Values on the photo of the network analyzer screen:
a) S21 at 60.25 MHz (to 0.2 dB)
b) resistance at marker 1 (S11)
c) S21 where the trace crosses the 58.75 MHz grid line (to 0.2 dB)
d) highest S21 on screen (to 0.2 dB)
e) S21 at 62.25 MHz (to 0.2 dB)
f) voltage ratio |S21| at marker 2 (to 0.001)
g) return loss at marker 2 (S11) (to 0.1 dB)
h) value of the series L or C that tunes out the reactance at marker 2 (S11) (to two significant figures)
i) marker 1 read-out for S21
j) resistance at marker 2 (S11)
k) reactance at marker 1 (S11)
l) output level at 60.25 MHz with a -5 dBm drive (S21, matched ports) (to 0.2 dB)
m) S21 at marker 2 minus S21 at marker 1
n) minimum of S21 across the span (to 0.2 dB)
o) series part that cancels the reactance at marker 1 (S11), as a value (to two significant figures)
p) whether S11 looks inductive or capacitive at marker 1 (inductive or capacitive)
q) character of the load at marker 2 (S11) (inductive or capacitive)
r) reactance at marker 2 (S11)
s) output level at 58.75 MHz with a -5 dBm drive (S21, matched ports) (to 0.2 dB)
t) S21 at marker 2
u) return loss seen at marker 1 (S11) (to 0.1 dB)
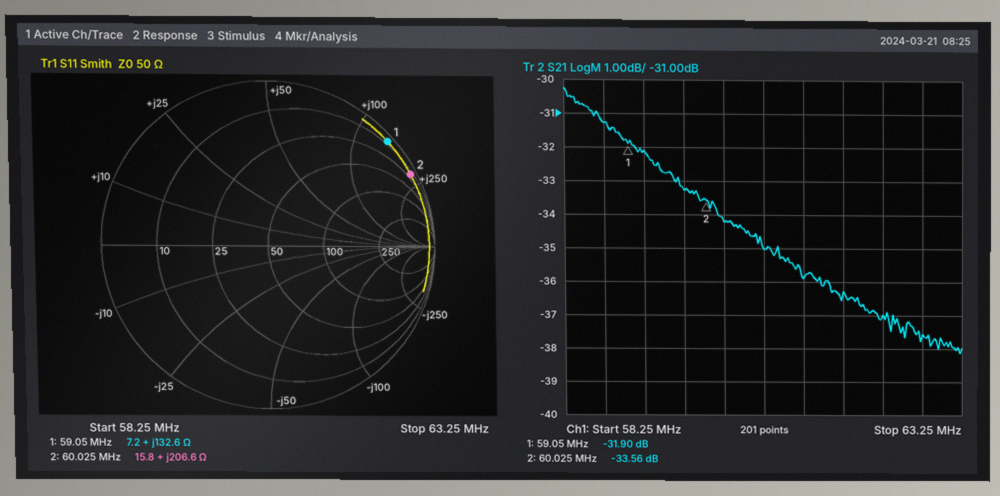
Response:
-34.2 dB
7.2 Ω
-31.2 dB
-30.2 dB
-37.0 dB
0.021
0.3 dB
13 pF
-31.90 dB
15.8 Ω
+132.6 Ω
-39.2 dBm
-1.66 dB
-38.2 dB
20 pF
inductive
inductive
+206.6 Ω
-36.2 dBm
-33.56 dB
0.3 dB
